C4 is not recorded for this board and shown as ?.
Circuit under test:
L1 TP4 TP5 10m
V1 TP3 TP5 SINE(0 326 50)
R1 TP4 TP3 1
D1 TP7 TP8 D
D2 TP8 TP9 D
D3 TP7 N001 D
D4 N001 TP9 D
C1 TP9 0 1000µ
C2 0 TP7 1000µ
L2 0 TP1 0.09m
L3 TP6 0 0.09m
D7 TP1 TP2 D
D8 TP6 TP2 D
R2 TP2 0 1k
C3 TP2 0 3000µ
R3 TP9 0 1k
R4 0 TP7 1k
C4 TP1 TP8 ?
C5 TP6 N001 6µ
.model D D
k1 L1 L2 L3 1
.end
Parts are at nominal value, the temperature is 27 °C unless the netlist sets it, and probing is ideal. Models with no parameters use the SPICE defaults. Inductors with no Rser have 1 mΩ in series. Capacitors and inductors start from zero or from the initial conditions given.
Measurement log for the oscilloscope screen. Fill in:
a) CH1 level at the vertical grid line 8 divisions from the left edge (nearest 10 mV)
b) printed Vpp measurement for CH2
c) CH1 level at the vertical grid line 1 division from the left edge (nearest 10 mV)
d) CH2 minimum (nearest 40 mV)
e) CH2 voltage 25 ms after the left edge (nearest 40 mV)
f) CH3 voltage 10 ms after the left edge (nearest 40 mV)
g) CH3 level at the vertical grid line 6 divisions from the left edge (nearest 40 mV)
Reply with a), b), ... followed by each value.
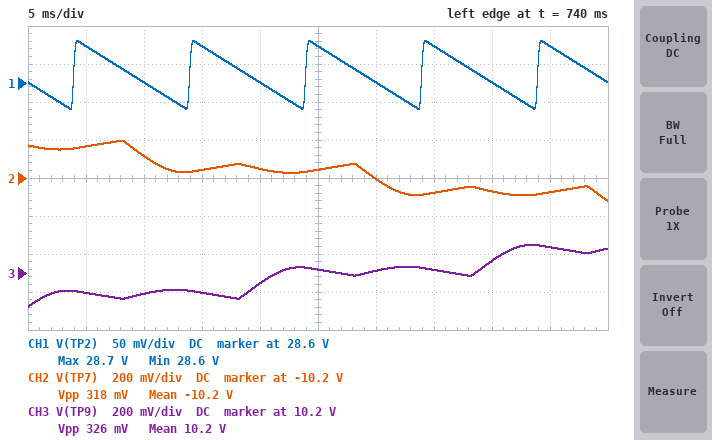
a) 28.60 V
b) 318 mV
c) 28.65 V
d) -10.32 V
e) -10.16 V
f) 10.08 V
g) 10.20 V
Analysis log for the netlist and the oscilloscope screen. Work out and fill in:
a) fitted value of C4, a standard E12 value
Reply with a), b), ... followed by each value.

a) 2.7 µF
